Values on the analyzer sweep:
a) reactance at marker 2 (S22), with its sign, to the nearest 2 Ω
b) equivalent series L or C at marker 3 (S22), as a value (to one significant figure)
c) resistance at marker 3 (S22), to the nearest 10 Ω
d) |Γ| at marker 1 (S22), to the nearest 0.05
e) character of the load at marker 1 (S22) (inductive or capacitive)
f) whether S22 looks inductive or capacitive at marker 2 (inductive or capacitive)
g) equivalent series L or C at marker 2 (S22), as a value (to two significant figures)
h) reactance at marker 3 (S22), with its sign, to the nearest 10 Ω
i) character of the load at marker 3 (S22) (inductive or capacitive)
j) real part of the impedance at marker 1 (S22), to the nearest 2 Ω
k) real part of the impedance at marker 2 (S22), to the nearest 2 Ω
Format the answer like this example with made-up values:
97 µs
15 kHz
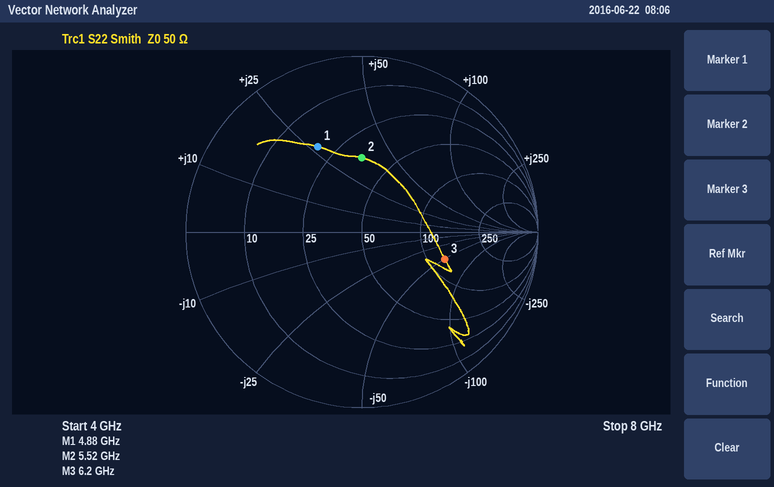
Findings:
+36 Ω
500 fF
120 Ω
0.55
inductive
inductive
1.0 nH
-50 Ω
capacitive
20 Ω
34 Ω
